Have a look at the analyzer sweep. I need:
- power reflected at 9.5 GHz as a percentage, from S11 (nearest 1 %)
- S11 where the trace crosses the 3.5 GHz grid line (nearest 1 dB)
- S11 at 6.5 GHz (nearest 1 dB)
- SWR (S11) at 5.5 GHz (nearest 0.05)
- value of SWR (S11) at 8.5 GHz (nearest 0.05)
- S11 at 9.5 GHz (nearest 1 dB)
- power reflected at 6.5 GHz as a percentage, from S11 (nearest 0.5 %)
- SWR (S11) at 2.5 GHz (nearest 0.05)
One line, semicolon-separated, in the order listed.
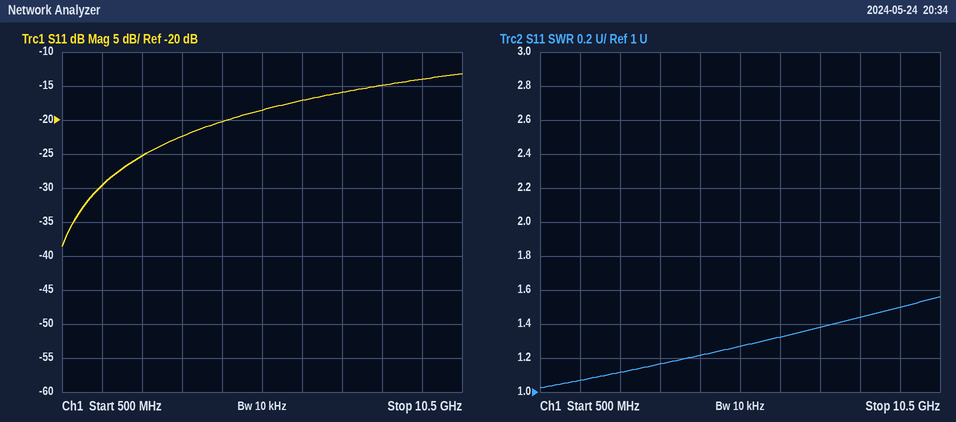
4 %; -22 dB; -17 dB; 1.25; 1.45; -14 dB; 2.0 %; 1.10
